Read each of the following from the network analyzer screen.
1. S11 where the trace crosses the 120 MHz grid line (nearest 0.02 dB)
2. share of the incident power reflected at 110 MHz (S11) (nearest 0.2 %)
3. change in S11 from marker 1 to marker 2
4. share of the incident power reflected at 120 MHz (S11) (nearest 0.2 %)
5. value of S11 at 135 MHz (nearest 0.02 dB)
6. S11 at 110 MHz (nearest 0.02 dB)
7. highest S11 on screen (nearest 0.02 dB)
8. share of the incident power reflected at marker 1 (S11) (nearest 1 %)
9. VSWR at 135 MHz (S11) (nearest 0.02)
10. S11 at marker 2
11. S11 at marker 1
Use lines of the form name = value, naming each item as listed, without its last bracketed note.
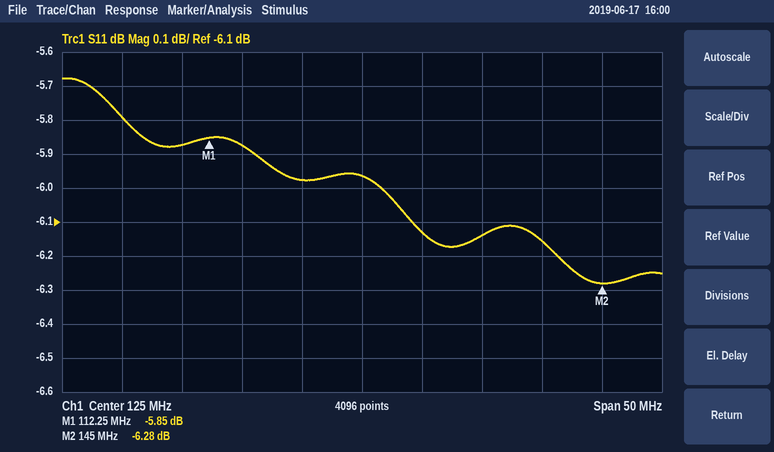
S11 where the trace crosses the 120 MHz grid line = -5.98 dB
share of the incident power reflected at 110 MHz (S11) = 25.8 %
change in S11 from marker 1 to marker 2 = -0.43 dB
share of the incident power reflected at 120 MHz (S11) = 25.2 %
value of S11 at 135 MHz = -6.14 dB
S11 at 110 MHz = -5.88 dB
highest S11 on screen = -5.68 dB
share of the incident power reflected at marker 1 (S11) = 26 %
VSWR at 135 MHz (S11) = 2.94
S11 at marker 2 = -6.28 dB
S11 at marker 1 = -5.85 dB
